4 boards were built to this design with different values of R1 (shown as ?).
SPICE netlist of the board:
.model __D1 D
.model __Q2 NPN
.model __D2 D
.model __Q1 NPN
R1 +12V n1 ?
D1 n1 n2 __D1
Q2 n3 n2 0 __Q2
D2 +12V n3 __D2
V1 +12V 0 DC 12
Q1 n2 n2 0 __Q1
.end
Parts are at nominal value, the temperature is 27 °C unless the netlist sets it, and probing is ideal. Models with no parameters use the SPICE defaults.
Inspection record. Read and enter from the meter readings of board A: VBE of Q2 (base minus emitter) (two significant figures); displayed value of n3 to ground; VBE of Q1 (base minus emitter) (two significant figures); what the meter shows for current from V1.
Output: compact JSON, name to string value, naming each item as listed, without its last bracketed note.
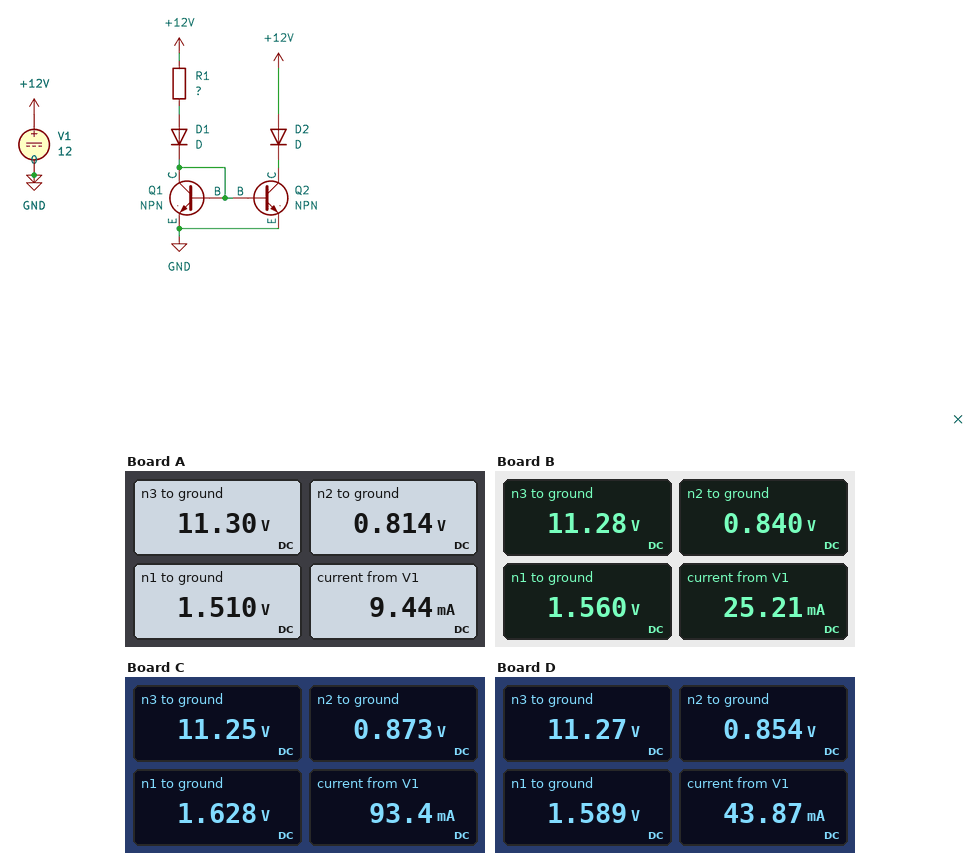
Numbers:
{"VBE of Q2 (base minus emitter)": "810 mV", "displayed value of n3 to ground": "11.30 V", "VBE of Q1 (base minus emitter)": "810 mV", "what the meter shows for current from V1": "9.44 mA"}
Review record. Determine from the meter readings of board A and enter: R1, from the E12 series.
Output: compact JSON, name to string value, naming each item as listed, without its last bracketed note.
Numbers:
{"R1, from the E12 series": "2.2 kΩ"}
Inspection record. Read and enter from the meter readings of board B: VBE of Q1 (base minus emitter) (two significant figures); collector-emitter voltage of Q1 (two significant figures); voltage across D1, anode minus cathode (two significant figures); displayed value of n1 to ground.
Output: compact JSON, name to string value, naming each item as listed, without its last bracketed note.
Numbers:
{"VBE of Q1 (base minus emitter)": "840 mV", "collector-emitter voltage of Q1": "840 mV", "voltage across D1, anode minus cathode": "720 mV", "displayed value of n1 to ground": "1.560 V"}
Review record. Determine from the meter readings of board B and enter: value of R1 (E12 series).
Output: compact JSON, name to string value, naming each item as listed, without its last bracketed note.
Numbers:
{"value of R1": "820 Ω"}
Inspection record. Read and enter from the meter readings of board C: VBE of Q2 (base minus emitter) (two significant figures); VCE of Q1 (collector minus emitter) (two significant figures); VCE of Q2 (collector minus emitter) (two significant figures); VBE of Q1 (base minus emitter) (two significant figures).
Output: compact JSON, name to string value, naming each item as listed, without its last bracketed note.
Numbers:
{"VBE of Q2 (base minus emitter)": "870 mV", "VCE of Q1 (collector minus emitter)": "870 mV", "VCE of Q2 (collector minus emitter)": "11 V", "VBE of Q1 (base minus emitter)": "870 mV"}
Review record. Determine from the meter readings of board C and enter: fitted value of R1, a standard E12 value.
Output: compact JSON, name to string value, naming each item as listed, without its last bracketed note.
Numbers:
{"fitted value of R1, a standard E12 value": "220 Ω"}
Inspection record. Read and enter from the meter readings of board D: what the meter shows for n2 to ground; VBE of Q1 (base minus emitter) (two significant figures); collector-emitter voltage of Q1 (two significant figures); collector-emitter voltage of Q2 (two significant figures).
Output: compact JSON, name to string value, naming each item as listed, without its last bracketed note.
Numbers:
{"what the meter shows for n2 to ground": "0.854 V", "VBE of Q1 (base minus emitter)": "850 mV", "collector-emitter voltage of Q1": "850 mV", "collector-emitter voltage of Q2": "11 V"}
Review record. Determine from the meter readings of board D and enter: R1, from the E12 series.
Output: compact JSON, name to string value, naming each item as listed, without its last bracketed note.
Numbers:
{"R1, from the E12 series": "470 Ω"}
